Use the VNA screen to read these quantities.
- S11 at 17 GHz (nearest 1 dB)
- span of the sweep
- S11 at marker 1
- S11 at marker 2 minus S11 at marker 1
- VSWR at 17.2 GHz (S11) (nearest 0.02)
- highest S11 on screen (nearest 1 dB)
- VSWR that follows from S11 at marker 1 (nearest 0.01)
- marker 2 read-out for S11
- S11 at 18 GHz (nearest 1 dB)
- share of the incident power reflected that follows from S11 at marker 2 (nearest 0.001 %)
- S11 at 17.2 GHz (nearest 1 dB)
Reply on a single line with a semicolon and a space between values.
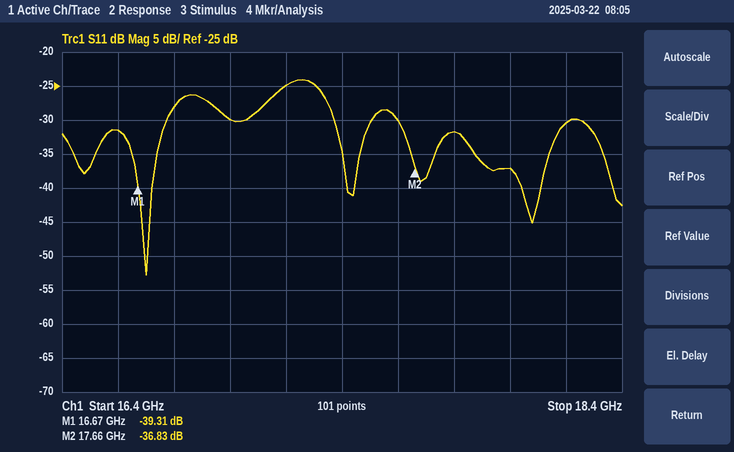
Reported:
-30 dB; 2 GHz; -39.31 dB; 2.48 dB; 1.12; -24 dB; 1.02; -36.83 dB; -37 dB; 0.021 %; -25 dB
